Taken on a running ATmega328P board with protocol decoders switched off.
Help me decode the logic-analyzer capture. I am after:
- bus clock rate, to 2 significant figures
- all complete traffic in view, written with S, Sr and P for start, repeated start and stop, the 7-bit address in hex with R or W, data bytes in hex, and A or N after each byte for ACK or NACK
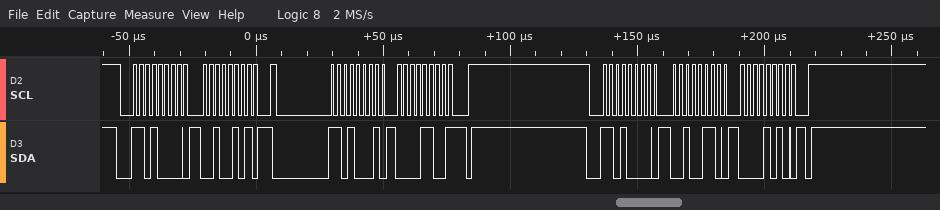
400 kHz
S 68W A 25 A Sr 68R A 0C N P S 68W A 26 A 0A A P
